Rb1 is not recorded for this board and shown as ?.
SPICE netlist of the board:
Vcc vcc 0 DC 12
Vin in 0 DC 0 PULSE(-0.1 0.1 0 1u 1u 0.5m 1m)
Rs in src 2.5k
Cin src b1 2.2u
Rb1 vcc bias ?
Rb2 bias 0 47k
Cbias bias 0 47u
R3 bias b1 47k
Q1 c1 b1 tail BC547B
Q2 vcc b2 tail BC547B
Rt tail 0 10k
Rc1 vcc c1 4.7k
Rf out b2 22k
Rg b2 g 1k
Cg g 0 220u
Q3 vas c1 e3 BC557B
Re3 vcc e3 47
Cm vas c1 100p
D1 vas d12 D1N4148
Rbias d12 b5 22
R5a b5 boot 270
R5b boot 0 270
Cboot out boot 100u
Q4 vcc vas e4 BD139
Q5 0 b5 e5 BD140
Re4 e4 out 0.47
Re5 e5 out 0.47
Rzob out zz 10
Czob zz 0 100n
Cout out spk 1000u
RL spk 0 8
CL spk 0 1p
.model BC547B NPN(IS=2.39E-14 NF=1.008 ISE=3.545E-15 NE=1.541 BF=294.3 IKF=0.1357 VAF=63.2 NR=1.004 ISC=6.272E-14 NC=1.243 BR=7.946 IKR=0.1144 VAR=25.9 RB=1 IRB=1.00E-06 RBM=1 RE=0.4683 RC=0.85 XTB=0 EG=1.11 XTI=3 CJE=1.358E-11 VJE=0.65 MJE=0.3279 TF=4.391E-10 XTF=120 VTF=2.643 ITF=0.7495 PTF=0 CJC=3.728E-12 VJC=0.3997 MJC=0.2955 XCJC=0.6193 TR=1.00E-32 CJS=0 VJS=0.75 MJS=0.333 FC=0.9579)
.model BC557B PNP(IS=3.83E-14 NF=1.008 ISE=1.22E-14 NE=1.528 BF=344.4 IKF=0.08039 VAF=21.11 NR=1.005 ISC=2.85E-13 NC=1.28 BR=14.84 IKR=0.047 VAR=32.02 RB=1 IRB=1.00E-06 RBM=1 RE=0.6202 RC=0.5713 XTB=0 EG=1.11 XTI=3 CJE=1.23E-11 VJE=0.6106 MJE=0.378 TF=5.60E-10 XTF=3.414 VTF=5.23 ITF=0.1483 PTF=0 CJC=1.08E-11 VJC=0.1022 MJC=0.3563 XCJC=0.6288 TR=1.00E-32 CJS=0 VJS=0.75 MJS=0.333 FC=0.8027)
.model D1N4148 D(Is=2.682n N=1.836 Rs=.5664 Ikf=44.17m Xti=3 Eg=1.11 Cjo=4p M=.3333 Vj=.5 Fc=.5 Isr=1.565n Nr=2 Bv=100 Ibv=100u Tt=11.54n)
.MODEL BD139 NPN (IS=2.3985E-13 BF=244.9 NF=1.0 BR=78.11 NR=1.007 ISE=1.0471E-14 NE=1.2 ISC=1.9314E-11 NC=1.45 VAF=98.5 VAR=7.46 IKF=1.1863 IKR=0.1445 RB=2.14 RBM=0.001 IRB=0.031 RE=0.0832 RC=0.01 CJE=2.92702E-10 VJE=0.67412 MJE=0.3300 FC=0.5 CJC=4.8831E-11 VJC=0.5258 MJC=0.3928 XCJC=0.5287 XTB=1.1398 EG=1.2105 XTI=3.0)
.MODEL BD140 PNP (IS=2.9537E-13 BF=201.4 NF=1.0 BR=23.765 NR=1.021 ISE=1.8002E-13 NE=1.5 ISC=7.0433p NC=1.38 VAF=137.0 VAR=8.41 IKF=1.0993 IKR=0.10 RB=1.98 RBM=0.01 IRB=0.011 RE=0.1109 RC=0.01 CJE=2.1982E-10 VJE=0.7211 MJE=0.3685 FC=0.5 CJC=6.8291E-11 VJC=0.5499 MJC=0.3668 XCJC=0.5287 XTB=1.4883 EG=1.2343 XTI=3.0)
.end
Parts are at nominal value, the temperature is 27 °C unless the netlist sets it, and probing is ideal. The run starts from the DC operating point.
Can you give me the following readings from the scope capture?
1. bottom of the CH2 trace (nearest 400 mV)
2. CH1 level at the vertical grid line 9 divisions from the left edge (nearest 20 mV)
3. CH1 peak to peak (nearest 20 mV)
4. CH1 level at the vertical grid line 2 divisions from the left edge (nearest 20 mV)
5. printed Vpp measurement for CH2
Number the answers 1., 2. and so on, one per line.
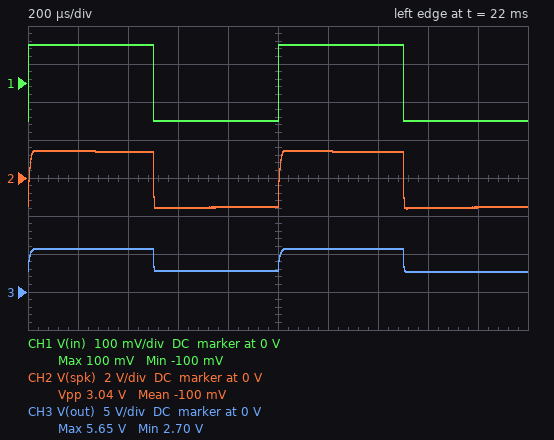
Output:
1. -1.6 V
2. -100 mV
3. 200 mV
4. 100 mV
5. 3.04 V
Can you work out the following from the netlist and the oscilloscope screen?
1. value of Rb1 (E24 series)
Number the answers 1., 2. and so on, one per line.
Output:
1. 130 kΩ
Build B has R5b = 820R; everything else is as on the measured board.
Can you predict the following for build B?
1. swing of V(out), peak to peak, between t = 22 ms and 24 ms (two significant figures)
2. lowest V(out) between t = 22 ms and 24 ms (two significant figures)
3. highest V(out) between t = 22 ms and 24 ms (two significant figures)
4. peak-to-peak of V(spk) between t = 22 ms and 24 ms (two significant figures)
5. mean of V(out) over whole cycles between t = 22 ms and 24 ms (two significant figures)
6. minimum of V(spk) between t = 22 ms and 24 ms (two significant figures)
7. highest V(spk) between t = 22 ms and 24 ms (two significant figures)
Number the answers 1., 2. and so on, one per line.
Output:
1. 3.5 V
2. 2.9 V
3. 6.4 V
4. 3.6 V
5. 4.6 V
6. -1.8 V
7. 1.7 V
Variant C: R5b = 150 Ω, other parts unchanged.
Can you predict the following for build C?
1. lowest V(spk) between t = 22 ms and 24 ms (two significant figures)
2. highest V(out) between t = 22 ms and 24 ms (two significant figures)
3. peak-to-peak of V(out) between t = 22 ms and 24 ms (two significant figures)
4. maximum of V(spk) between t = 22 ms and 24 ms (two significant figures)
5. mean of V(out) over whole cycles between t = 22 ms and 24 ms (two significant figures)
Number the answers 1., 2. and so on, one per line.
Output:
1. -1.1 V
2. 4.8 V
3. 2.1 V
4. 1.0 V
5. 3.7 V
